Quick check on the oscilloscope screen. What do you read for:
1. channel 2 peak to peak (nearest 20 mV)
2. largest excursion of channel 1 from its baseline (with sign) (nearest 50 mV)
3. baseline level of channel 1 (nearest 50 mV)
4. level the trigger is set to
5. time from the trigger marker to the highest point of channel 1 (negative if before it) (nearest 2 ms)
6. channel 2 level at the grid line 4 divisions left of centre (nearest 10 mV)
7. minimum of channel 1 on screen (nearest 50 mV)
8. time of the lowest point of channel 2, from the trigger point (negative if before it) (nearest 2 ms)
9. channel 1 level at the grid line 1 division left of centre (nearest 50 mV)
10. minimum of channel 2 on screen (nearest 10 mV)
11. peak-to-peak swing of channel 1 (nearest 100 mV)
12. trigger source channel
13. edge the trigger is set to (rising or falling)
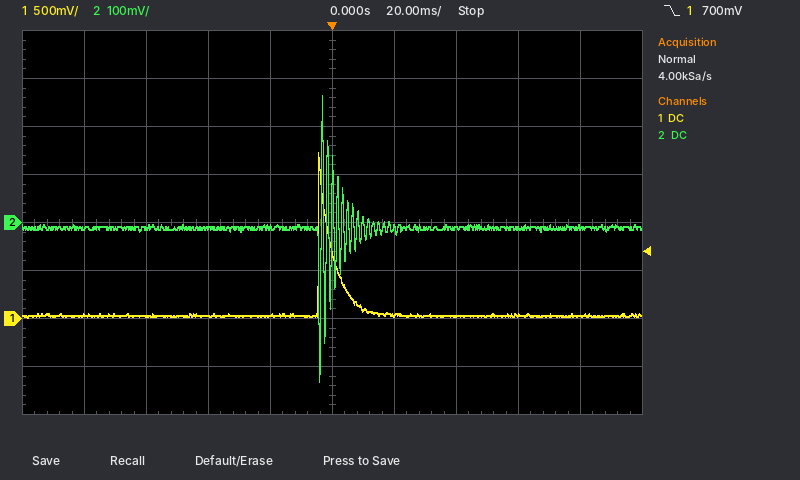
600 mV
+1.70 V
50 mV
700 mV
-4 ms
-10 mV
0 mV
-4 ms
50 mV
-330 mV
1.70 V
channel 1
falling
